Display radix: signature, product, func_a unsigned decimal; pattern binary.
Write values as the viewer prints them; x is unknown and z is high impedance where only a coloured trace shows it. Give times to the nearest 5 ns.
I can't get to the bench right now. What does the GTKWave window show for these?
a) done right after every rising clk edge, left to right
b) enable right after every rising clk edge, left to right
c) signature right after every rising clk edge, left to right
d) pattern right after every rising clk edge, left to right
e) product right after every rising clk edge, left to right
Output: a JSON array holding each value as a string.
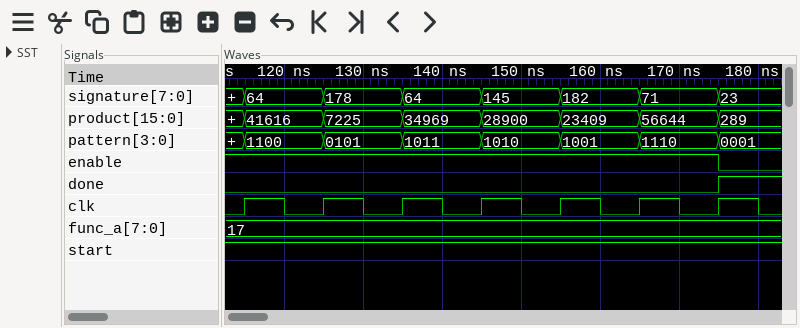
["0 0 0 0 0 0 1", "1 1 1 1 1 1 0", "64, 178, 64, 145, 182, 71, 23", "1100, 0101, 1011, 1010, 1001, 1110, 0001", "41616, 7225, 34969, 28900, 23409, 56644, 289"]
